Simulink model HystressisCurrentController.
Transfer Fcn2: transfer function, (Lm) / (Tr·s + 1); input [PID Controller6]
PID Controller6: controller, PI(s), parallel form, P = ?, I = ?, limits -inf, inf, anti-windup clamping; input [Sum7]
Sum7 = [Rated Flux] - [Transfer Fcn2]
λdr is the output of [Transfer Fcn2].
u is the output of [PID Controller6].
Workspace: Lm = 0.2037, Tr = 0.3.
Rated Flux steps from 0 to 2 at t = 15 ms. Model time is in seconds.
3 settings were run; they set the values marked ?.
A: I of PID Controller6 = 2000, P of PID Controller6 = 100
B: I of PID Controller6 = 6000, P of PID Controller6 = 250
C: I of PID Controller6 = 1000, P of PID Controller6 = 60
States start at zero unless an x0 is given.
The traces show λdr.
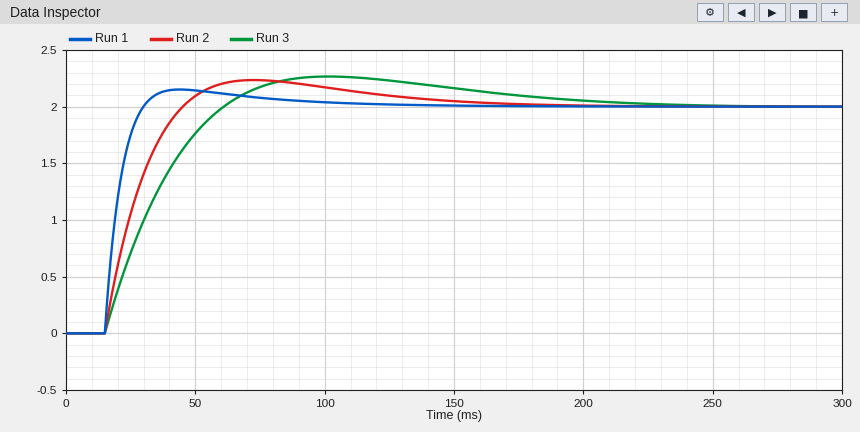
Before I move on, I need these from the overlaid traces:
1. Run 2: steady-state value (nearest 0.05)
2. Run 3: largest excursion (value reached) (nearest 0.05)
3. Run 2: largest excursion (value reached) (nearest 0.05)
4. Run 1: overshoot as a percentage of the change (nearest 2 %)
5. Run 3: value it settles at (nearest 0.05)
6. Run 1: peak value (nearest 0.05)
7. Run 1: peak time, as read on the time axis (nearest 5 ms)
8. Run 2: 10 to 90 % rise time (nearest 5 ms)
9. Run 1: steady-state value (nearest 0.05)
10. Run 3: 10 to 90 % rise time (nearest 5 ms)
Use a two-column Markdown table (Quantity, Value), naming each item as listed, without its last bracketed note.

| Quantity | Value |
|---|---|
| Run 2: steady-state value | 2.00 |
| Run 3: largest excursion (value reached) | 2.25 |
| Run 2: largest excursion (value reached) | 2.25 |
| Run 1: overshoot as a percentage of the change | 8 % |
| Run 3: value it settles at | 2.00 |
| Run 1: peak value | 2.15 |
| Run 1: peak time, as read on the time axis | 45 ms |
| Run 2: 10 to 90 % rise time | 20 ms |
| Run 1: steady-state value | 2.00 |
| Run 3: 10 to 90 % rise time | 35 ms |
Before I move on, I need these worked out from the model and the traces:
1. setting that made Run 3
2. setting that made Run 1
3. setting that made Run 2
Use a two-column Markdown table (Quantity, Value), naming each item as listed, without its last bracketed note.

| Quantity | Value |
|---|---|
| setting that made Run 3 | C |
| setting that made Run 1 | B |
| setting that made Run 2 | A |
